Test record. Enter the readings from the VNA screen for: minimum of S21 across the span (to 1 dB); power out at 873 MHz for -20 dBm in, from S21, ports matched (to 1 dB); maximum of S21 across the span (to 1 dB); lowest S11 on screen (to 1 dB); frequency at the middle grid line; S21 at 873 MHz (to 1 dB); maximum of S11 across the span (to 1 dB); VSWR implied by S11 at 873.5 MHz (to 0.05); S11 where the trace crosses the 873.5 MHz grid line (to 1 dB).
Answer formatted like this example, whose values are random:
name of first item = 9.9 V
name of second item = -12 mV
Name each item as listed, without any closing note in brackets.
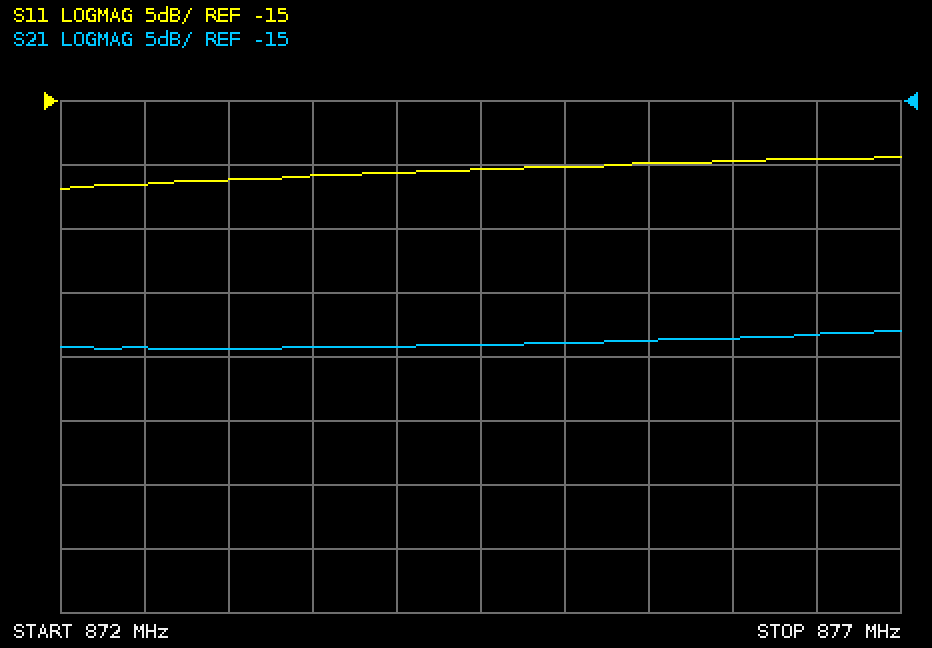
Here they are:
minimum of S21 across the span = -34 dB
power out at 873 MHz for -20 dBm in, from S21, ports matched = -54 dBm
maximum of S21 across the span = -33 dB
lowest S11 on screen = -22 dB
frequency at the middle grid line = 874.5 MHz
S21 at 873 MHz = -34 dB
maximum of S11 across the span = -19 dB
VSWR implied by S11 at 873.5 MHz = 1.20
S11 where the trace crosses the 873.5 MHz grid line = -21 dB
